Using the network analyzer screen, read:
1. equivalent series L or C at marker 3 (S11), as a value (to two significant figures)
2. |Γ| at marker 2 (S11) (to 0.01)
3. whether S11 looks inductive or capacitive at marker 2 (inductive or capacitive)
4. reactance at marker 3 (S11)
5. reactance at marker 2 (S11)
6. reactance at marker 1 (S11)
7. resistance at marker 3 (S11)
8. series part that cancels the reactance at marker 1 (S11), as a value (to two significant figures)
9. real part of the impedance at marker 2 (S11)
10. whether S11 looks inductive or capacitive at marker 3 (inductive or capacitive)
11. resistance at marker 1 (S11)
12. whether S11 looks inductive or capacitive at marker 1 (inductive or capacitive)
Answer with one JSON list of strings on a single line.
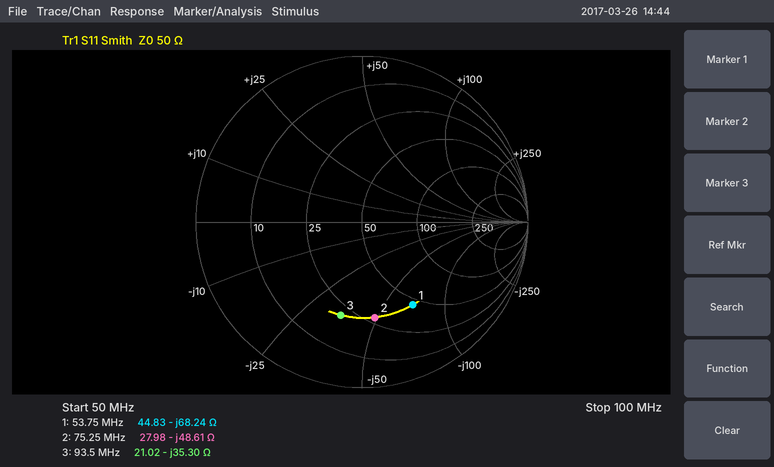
["48 pF", "0.58", "capacitive", "-35.30 Ω", "-48.61 Ω", "-68.24 Ω", "21.02 Ω", "200 nH", "27.98 Ω", "capacitive", "44.83 Ω", "capacitive"]
